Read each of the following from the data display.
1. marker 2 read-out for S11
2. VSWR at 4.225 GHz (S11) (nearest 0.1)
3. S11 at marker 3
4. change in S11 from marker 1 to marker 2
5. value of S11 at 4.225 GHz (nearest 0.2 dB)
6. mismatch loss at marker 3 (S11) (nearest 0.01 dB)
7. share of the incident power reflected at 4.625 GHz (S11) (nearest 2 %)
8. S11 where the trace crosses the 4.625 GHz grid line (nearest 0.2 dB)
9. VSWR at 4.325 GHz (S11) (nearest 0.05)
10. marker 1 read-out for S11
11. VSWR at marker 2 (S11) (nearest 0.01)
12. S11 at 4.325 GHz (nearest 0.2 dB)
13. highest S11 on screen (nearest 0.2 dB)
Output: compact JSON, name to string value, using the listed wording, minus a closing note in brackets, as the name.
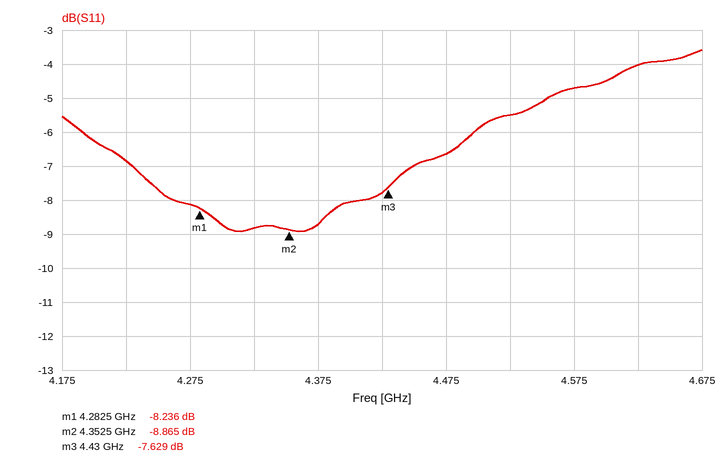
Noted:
{"marker 2 read-out for S11": "-8.865 dB", "VSWR at 4.225 GHz (S11)": "2.7", "S11 at marker 3": "-7.629 dB", "change in S11 from marker 1 to marker 2": "-0.629 dB", "value of S11 at 4.225 GHz": "-6.8 dB", "mismatch loss at marker 3 (S11)": "0.82 dB", "share of the incident power reflected at 4.625 GHz (S11)": "40 %", "S11 where the trace crosses the 4.625 GHz grid line": "-4.0 dB", "VSWR at 4.325 GHz (S11)": "2.15", "marker 1 read-out for S11": "-8.236 dB", "VSWR at marker 2 (S11)": "2.13", "S11 at 4.325 GHz": "-8.8 dB", "highest S11 on screen": "-3.6 dB"}
